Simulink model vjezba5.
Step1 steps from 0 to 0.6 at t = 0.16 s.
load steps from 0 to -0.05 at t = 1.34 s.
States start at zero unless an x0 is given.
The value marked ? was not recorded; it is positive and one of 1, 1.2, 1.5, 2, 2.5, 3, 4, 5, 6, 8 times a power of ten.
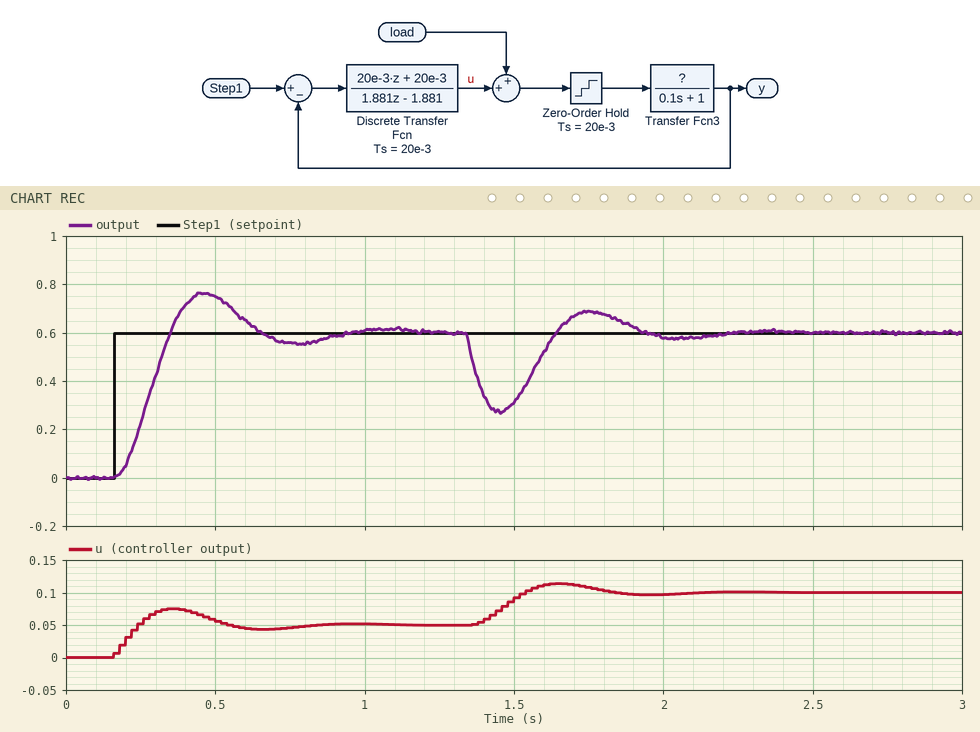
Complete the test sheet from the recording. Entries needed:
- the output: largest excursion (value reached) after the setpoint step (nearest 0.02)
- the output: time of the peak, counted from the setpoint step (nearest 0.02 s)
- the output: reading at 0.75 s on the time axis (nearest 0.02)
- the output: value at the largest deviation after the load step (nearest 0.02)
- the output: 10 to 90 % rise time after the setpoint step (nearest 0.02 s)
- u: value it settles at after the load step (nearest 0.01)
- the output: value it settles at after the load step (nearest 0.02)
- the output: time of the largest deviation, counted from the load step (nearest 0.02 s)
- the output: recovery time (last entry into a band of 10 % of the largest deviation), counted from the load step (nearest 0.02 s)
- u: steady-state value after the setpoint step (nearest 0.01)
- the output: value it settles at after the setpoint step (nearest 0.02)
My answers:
0.76
0.30 s
0.56
0.28
0.12 s
0.10
0.60
0.12 s
0.54 s
0.05
0.60
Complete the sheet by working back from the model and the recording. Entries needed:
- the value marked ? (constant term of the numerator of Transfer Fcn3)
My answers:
12
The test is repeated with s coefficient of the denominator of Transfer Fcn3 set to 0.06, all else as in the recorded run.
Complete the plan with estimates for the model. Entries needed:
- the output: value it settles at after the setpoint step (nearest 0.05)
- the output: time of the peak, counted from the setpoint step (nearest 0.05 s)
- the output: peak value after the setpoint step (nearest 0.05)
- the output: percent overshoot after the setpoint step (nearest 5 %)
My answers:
0.60
0.25 s
0.70
15 %
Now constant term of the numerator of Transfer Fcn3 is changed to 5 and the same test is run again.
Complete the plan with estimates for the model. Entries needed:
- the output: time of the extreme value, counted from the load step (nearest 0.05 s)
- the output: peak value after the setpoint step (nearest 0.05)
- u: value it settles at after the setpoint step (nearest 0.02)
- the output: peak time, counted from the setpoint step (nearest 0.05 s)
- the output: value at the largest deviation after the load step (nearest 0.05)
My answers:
0.15 s
0.65
0.12
0.55 s
0.45
